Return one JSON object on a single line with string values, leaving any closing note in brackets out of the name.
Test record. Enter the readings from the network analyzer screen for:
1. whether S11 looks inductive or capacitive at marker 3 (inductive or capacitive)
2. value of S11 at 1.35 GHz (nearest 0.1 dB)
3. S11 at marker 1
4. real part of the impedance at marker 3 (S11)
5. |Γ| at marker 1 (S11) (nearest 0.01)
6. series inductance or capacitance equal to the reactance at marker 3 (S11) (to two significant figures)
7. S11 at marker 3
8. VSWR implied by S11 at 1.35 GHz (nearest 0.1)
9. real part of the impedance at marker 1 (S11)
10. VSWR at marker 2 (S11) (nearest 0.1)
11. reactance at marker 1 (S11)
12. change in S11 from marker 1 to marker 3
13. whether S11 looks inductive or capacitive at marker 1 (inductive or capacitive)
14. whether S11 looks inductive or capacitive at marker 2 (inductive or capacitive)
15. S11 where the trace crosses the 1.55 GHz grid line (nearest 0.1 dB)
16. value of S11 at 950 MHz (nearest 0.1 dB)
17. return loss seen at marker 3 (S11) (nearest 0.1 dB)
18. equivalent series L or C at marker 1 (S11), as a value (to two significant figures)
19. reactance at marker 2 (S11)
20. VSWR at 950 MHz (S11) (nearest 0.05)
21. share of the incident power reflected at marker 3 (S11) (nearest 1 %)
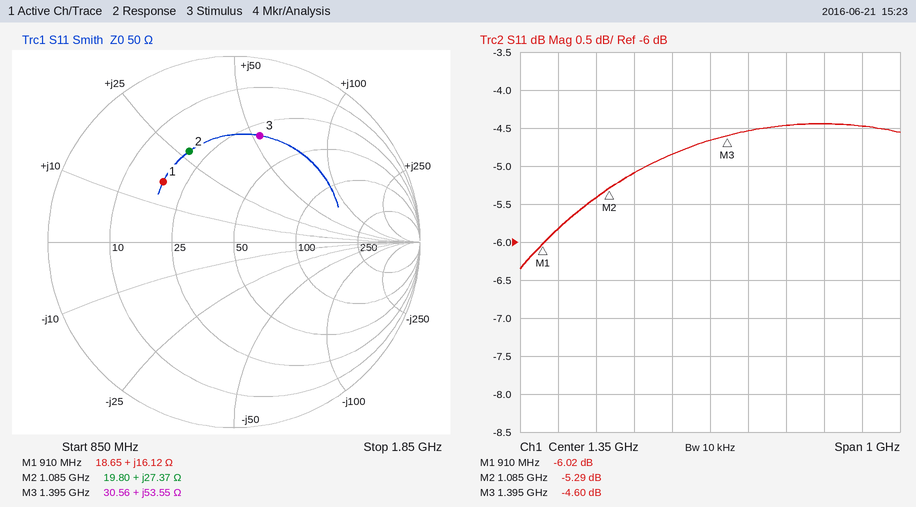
{"whether S11 looks inductive or capacitive at marker 3": "inductive", "value of S11 at 1.35 GHz": "-4.7 dB", "S11 at marker 1": "-6.02 dB", "real part of the impedance at marker 3": "30.56 Ω", "|Γ| at marker 1 (S11)": "0.50", "series inductance or capacitance equal to the reactance at marker 3 (S11)": "6.1 nH", "S11 at marker 3": "-4.60 dB", "VSWR implied by S11 at 1.35 GHz": "3.8", "real part of the impedance at marker 1": "18.65 Ω", "VSWR at marker 2 (S11)": "3.4", "reactance at marker 1": "+16.12 Ω", "change in S11 from marker 1 to marker 3": "1.42 dB", "whether S11 looks inductive or capacitive at marker 1": "inductive", "whether S11 looks inductive or capacitive at marker 2": "inductive", "S11 where the trace crosses the 1.55 GHz grid line": "-4.5 dB", "value of S11 at 950 MHz": "-5.8 dB", "return loss seen at marker 3 (S11)": "4.6 dB", "equivalent series L or C at marker 1 (S11), as a value": "2.8 nH", "reactance at marker 2": "+27.37 Ω", "VSWR at 950 MHz (S11)": "3.10", "share of the incident power reflected at marker 3 (S11)": "35 %"}
